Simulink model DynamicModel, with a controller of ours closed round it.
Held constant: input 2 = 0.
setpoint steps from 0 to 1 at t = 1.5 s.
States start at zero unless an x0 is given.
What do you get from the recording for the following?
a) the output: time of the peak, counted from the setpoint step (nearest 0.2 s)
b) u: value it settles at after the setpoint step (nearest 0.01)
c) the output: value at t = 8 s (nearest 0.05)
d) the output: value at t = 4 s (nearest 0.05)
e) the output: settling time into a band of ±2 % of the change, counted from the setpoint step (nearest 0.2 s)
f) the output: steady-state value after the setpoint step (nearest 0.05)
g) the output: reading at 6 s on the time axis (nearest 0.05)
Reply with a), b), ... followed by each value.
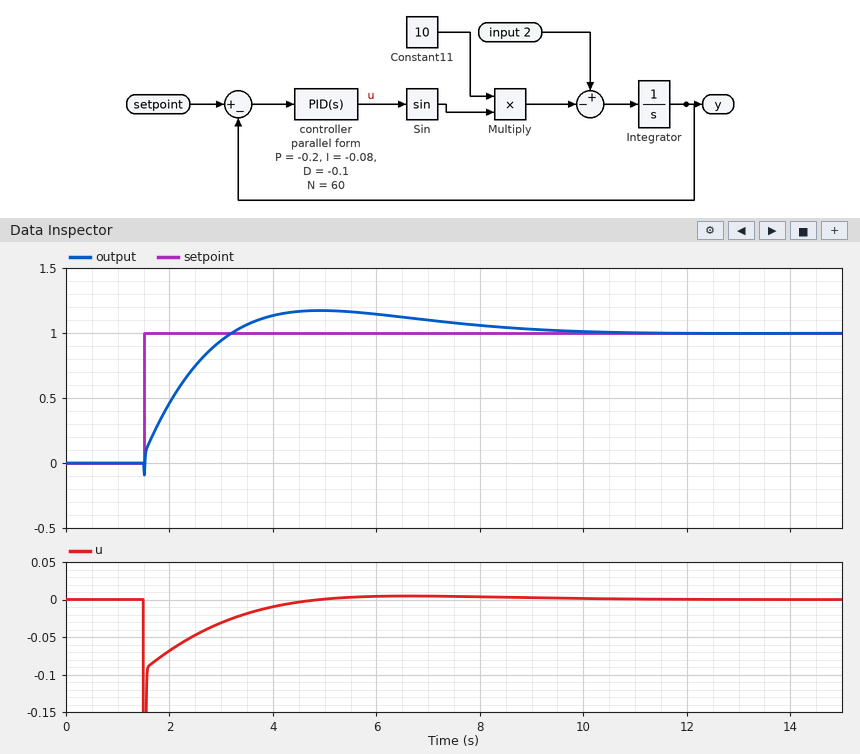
a) 3.4 s
b) 0.00
c) 1.05
d) 1.15
e) 8.0 s
f) 1.00
g) 1.15
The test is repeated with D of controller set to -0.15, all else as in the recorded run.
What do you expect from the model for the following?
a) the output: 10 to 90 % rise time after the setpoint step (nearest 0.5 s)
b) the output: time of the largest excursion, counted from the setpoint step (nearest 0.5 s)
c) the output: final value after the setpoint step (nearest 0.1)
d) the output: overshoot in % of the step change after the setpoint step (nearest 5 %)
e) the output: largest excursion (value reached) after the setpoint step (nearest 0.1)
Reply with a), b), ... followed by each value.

a) 1.5 s
b) 4.0 s
c) 1.0
d) 20 %
e) 1.2
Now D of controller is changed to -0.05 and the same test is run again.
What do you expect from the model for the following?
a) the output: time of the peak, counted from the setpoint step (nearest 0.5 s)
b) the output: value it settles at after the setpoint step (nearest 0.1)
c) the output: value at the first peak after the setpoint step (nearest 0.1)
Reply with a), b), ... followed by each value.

a) 3.0 s
b) 1.0
c) 1.1
